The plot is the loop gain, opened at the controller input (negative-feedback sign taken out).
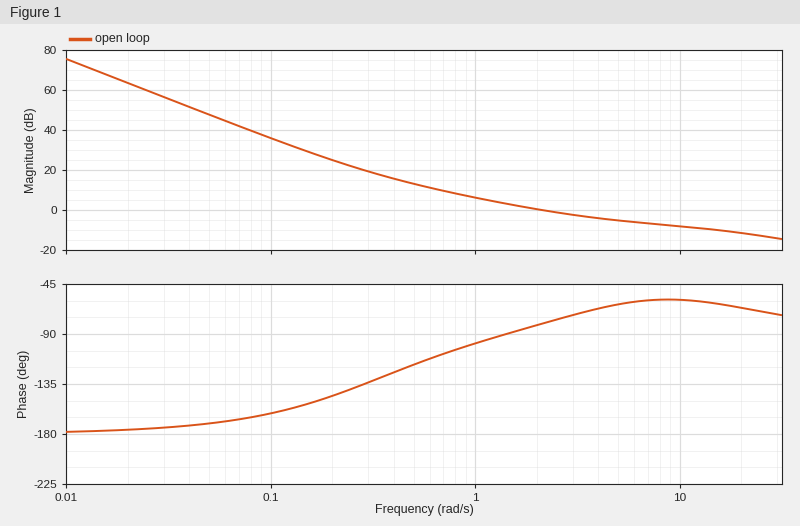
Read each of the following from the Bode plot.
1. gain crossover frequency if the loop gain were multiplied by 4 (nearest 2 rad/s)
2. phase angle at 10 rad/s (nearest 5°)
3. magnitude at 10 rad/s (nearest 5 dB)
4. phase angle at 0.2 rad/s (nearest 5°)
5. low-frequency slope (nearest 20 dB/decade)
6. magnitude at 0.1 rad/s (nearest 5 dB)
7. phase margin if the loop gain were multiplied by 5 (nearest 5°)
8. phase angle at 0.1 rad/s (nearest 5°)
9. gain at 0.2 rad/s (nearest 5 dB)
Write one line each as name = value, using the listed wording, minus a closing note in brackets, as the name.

gain crossover frequency if the loop gain were multiplied by 4 = 22 rad/s
phase angle at 10 rad/s = -60°
magnitude at 10 rad/s = -10 dB
phase angle at 0.2 rad/s = -145°
low-frequency slope = -40 dB/decade
magnitude at 0.1 rad/s = 35 dB
phase margin if the loop gain were multiplied by 5 = 110°
phase angle at 0.1 rad/s = -160°
gain at 0.2 rad/s = 25 dB
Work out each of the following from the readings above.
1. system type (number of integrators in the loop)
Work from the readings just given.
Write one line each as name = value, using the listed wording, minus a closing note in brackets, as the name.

system type = 2
